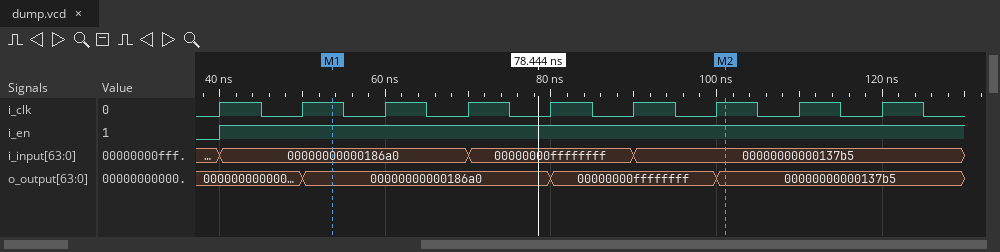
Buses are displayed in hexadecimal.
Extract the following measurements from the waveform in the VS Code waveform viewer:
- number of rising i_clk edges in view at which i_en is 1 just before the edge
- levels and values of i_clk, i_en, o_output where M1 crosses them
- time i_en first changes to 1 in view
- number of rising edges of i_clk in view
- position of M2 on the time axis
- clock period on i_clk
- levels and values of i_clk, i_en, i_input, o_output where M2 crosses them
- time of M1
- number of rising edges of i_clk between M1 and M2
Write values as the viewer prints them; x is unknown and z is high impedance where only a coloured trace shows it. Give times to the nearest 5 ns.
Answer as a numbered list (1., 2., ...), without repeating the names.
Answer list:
1. 8
2. i_clk=1, i_en=1, o_output=00000000000186a0
3. 40 ns
4. 9
5. 100 ns
6. 10 ns
7. i_clk=1, i_en=1, i_input=00000000000137b5, o_output=00000000000137b5
8. 55 ns
9. 5
